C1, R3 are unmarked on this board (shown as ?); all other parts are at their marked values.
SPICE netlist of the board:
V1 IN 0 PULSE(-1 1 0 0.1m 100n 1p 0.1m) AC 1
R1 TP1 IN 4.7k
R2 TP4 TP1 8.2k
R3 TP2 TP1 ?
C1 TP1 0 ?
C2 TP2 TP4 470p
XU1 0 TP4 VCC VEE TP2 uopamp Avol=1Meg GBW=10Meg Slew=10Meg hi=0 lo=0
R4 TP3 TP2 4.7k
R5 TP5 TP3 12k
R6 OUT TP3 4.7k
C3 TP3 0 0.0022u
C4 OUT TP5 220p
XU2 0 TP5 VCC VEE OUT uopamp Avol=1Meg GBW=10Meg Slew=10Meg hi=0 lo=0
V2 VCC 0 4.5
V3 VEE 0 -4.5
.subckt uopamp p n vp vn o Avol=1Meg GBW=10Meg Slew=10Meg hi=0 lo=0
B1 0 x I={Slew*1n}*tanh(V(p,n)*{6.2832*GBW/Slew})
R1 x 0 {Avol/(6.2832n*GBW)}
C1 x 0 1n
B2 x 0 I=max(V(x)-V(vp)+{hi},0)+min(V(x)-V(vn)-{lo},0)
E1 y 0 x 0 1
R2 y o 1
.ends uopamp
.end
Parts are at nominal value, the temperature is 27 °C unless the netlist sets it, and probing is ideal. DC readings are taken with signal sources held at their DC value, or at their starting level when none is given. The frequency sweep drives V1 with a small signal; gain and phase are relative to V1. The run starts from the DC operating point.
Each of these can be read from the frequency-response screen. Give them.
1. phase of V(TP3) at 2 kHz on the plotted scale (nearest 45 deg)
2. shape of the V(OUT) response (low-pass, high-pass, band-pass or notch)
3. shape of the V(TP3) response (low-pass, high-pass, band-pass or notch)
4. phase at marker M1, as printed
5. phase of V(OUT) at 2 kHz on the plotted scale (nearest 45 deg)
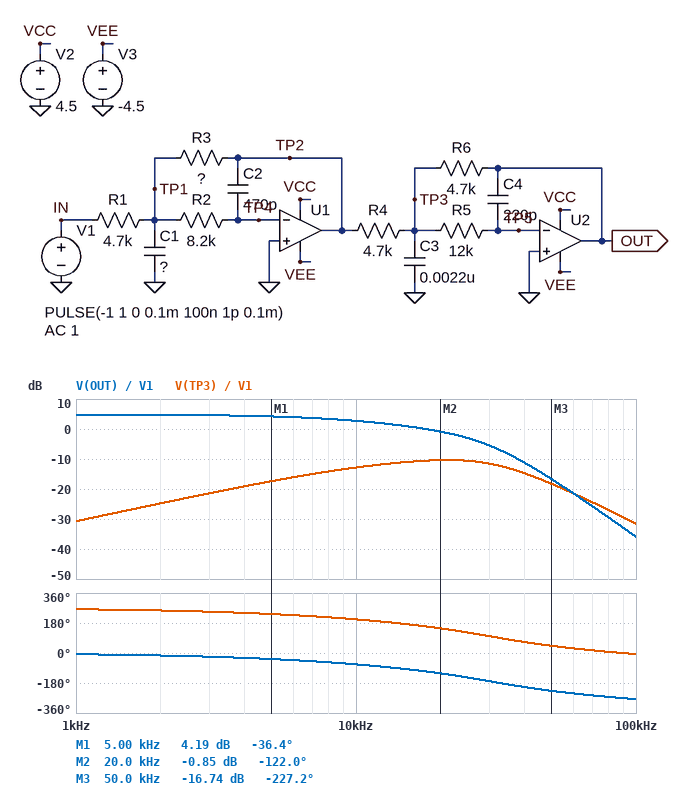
270 deg
low-pass
band-pass
-36.4 deg
0 deg
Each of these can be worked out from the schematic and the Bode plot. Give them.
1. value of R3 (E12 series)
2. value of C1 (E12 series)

8.2 kΩ
470 pF
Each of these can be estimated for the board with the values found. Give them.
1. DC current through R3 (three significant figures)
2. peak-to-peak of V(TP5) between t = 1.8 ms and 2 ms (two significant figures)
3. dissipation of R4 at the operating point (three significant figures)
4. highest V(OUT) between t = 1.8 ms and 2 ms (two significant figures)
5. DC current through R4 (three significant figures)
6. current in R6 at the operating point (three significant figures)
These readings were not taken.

213 µA
2.5 mV
648 µW
1.1 V
371 µA
371 µA
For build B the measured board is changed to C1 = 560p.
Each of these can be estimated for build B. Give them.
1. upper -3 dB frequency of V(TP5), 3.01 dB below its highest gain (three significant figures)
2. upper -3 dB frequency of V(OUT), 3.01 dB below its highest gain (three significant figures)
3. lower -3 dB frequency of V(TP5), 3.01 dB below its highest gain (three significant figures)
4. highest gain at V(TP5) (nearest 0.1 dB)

35.9 kHz
12.8 kHz
9.13 kHz
-54.7 dB
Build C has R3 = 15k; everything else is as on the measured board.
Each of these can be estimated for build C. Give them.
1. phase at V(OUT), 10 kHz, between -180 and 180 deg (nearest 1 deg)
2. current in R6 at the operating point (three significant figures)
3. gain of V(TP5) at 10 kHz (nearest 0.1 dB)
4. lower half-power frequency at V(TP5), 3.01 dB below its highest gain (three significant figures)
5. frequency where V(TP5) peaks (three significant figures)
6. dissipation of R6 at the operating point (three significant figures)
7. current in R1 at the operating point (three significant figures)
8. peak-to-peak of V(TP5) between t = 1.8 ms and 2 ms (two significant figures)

-83 deg
679 µA
-54.4 dB
6.47 kHz
19.1 kHz
2.17 mW
213 µA
3.3 mV
